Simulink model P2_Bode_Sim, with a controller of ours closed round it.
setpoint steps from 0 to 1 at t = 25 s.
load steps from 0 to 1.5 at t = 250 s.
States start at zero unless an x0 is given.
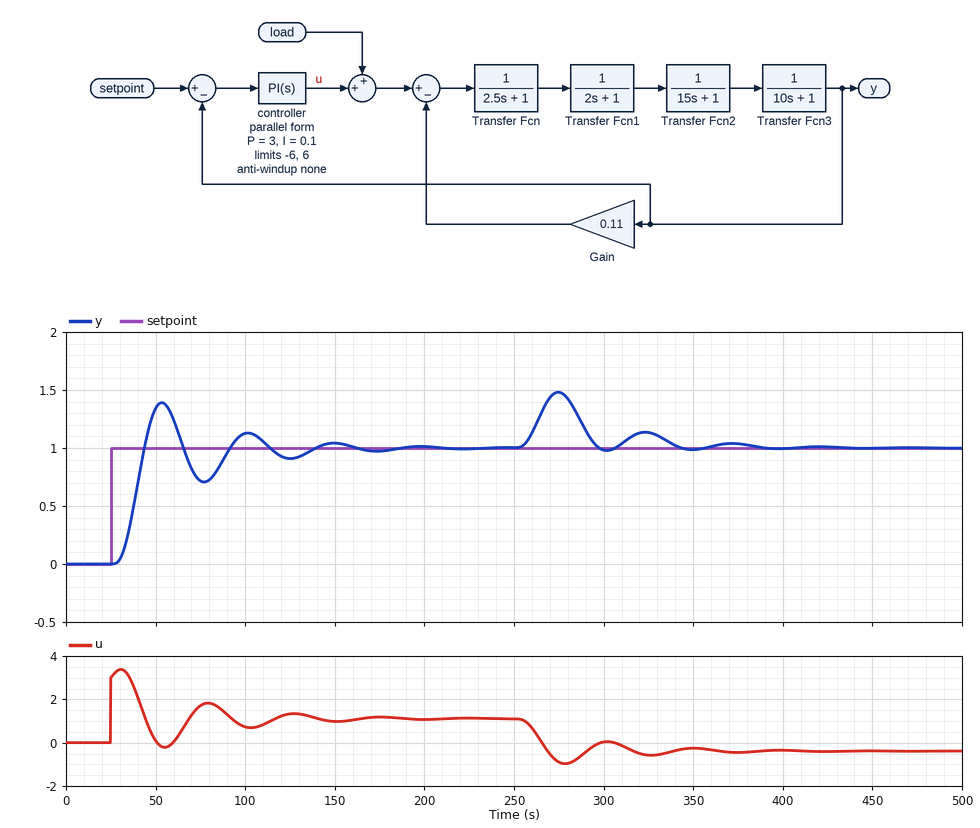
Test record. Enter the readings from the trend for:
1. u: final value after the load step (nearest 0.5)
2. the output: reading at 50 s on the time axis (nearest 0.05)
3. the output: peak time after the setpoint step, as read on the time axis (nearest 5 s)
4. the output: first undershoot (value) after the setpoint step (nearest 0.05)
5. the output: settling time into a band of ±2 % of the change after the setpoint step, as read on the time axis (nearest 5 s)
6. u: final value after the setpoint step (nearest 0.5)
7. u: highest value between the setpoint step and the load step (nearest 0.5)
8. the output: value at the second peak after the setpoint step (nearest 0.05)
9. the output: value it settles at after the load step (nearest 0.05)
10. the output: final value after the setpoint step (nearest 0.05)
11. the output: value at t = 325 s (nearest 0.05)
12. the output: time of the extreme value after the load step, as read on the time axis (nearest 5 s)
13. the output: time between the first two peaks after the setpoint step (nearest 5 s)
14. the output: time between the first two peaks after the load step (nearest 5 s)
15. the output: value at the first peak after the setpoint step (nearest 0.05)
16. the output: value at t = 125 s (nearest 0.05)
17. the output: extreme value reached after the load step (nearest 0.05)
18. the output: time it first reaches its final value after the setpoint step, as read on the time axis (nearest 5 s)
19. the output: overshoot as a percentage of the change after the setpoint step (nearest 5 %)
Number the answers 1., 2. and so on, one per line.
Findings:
1. -0.5
2. 1.35
3. 55 s
4. 0.70
5. 180 s
6. 1.0
7. 3.5
8. 1.15
9. 1.00
10. 1.00
11. 1.15
12. 275 s
13. 50 s
14. 50 s
15. 1.40
16. 0.90
17. 1.50
18. 45 s
19. 40 %
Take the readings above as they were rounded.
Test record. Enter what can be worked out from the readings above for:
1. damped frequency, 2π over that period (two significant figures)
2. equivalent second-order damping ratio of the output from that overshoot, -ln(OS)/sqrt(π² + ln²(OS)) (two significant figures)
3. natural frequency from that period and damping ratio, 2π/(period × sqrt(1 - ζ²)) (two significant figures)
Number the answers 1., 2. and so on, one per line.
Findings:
1. 0.13 rad/s
2. 0.28
3. 0.13 rad/s
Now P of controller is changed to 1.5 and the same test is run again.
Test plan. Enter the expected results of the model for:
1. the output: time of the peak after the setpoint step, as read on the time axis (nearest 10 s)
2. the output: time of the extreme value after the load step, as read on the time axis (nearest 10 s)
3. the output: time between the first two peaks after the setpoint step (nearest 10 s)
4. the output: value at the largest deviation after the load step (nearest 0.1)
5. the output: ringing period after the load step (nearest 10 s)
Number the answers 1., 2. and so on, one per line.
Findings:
1. 60 s
2. 280 s
3. 70 s
4. 1.6
5. 70 s
